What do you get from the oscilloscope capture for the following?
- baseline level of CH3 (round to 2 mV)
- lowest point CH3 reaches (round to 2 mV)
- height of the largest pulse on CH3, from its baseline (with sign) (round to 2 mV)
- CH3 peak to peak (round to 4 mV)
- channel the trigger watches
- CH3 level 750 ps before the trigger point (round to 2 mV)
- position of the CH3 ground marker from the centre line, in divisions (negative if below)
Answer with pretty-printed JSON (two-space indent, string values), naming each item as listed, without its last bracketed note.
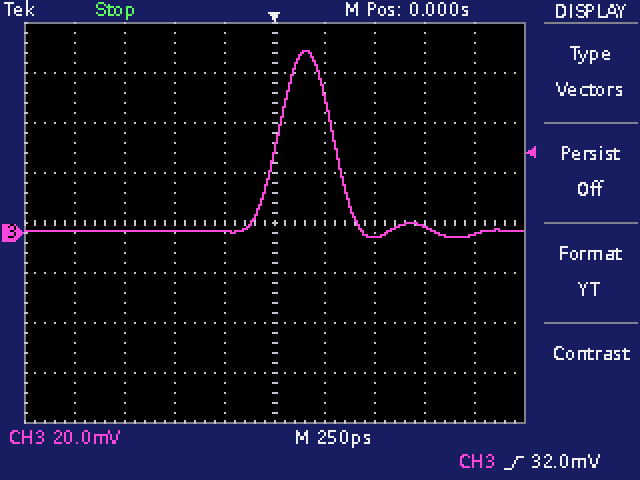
{
  "baseline level of CH3": "0 mV",
  "lowest point CH3 reaches": "-2 mV",
  "height of the largest pulse on CH3, from its baseline (with sign)": "+72 mV",
  "CH3 peak to peak": "76 mV",
  "channel the trigger watches": "CH3",
  "CH3 level 750 ps before the trigger point": "0 mV",
  "position of the CH3 ground marker from the centre line, in divisions": "-0.2 div"
}
